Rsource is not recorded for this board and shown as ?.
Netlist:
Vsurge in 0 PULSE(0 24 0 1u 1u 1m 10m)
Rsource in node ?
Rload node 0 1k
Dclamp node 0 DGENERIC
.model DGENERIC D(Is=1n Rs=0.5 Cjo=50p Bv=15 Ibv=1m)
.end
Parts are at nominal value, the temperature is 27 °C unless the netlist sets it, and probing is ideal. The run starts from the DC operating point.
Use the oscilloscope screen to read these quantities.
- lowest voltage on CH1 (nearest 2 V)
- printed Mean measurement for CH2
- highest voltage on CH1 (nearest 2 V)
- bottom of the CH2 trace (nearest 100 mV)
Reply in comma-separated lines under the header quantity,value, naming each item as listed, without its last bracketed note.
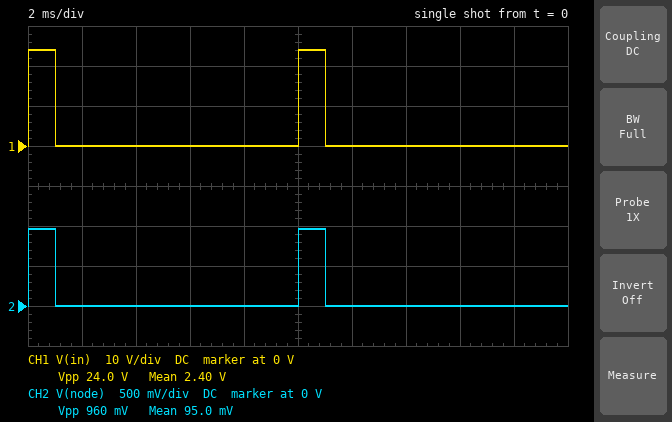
quantity,value
lowest voltage on CH1,0 V
printed Mean measurement for CH2,95.0 mV
highest voltage on CH1,24 V
bottom of the CH2 trace,0 V
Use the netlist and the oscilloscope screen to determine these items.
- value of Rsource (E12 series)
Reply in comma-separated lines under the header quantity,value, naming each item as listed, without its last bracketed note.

quantity,value
value of Rsource,27 Ω
